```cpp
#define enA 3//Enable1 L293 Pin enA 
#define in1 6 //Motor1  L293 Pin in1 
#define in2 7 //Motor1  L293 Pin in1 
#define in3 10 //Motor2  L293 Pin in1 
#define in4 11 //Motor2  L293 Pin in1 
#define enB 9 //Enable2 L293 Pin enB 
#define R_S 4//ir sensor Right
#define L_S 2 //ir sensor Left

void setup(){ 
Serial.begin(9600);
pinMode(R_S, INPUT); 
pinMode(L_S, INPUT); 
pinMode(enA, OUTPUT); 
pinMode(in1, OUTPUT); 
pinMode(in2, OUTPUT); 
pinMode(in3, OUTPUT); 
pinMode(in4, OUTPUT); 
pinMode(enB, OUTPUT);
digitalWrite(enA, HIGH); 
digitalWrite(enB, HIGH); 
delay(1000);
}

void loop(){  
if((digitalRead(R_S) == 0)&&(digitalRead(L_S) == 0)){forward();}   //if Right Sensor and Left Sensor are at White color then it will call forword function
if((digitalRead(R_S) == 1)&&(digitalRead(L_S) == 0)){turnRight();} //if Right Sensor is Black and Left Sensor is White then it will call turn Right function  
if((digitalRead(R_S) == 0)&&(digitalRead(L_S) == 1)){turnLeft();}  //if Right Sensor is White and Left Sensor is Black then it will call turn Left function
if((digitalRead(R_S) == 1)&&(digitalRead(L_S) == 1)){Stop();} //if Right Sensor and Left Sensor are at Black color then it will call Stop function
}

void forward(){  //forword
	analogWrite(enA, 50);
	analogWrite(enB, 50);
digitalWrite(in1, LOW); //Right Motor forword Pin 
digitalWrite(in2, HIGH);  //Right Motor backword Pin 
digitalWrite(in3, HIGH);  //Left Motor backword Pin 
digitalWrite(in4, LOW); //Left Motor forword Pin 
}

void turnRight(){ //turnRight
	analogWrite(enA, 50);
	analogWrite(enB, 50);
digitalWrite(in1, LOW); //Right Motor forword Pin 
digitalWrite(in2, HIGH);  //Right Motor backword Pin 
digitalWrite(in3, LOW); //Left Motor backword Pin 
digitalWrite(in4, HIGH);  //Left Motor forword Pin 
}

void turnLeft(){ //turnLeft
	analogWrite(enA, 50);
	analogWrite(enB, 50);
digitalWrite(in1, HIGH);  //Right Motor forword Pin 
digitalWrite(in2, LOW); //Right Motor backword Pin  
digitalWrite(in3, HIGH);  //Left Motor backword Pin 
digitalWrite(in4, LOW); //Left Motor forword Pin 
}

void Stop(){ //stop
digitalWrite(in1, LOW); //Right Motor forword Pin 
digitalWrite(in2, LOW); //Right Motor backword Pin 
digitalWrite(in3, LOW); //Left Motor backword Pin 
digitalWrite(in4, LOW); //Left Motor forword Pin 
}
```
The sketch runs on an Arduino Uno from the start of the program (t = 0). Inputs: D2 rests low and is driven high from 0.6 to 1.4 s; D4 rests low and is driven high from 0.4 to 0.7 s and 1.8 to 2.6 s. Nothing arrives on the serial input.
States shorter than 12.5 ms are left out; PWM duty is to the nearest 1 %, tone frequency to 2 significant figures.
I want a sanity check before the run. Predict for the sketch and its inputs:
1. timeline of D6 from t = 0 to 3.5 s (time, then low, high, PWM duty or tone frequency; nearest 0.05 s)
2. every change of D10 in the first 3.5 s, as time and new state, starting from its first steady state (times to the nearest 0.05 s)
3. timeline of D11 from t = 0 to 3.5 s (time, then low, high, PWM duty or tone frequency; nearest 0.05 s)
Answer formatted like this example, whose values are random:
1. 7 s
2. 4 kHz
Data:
1. 0 s low; 1 s high; 1.4 s low
2. 0 s low; 1 s high; 1.8 s low; 2.6 s high
3. 0 s low; 1.8 s high; 2.6 s low
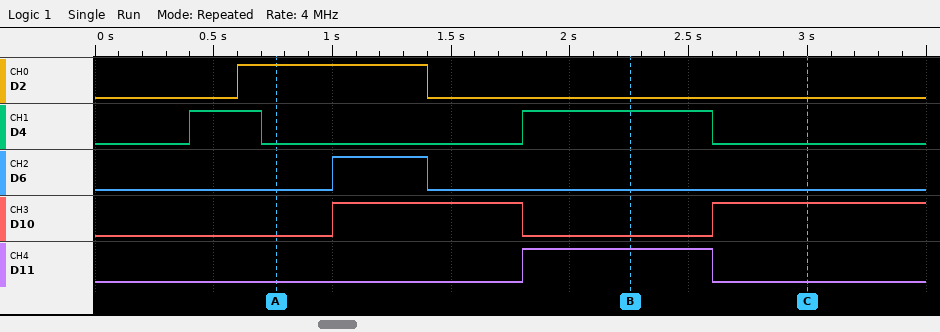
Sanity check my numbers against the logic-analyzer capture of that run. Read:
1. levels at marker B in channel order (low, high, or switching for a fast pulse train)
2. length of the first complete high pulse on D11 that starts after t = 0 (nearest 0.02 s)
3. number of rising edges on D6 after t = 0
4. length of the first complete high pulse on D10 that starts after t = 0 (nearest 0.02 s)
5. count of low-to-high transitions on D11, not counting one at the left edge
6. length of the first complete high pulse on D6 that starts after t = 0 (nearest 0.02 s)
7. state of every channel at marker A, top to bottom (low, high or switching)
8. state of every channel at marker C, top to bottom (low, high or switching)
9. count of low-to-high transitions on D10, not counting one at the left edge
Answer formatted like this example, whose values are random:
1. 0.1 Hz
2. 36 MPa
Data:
1. D2 low, D4 high, D6 low, D10 low, D11 high
2. 0.80 s
3. 1
4. 0.80 s
5. 1
6. 0.40 s
7. D2 high, D4 low, D6 low, D10 low, D11 low
8. D2 low, D4 low, D6 low, D10 high, D11 low
9. 2
